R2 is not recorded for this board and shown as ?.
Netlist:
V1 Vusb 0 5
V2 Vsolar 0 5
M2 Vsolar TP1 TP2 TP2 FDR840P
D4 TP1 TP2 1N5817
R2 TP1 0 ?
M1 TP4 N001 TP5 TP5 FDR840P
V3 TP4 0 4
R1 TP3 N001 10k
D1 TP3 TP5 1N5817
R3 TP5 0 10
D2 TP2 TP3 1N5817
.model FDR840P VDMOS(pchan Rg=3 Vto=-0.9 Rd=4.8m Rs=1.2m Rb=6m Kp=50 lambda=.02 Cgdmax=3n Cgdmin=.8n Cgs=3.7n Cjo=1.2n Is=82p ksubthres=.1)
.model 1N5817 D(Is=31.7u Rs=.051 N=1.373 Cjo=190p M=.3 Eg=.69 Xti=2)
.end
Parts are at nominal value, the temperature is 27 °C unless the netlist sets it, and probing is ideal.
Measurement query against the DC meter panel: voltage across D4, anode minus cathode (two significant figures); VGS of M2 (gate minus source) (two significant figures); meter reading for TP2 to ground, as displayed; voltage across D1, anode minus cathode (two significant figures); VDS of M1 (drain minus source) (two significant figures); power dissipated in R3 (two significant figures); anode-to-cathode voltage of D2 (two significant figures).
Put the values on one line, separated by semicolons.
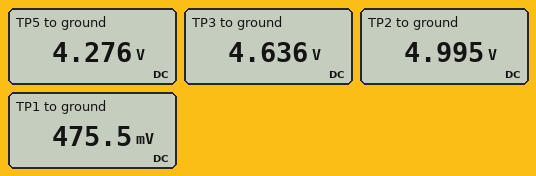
-4.5 V; -4.5 V; 4.995 V; 360 mV; -280 mV; 1.8 W; 360 mV
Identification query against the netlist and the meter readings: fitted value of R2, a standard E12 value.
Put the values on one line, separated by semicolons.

15 kΩ
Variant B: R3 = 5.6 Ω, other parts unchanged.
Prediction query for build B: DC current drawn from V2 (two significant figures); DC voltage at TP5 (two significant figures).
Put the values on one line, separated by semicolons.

750 mA; 4.2 V
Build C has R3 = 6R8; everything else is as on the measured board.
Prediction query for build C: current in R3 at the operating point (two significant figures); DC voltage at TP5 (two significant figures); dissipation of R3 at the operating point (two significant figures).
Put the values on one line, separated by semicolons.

620 mA; 4.2 V; 2.6 W
